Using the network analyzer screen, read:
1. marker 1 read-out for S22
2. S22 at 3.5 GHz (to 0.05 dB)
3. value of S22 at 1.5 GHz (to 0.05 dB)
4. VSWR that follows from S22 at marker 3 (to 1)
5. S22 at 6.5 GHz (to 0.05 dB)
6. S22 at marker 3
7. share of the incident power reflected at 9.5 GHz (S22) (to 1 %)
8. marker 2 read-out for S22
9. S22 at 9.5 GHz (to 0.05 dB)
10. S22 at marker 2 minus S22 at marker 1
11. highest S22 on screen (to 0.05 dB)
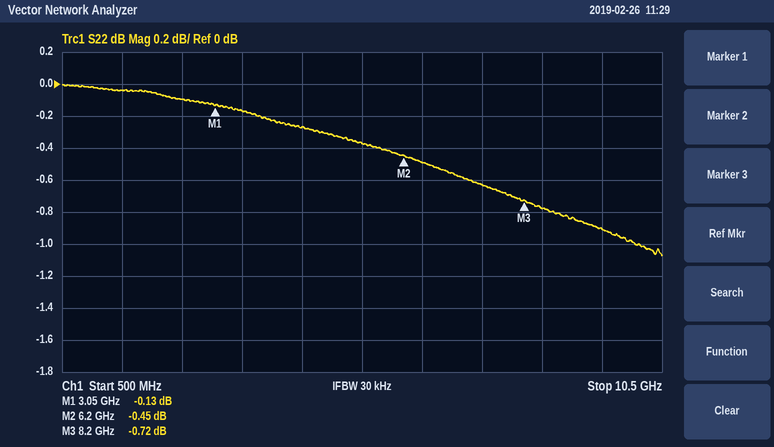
-0.13 dB
-0.15 dB
-0.05 dB
24
-0.50 dB
-0.72 dB
81 %
-0.45 dB
-0.90 dB
-0.32 dB
0.00 dB
